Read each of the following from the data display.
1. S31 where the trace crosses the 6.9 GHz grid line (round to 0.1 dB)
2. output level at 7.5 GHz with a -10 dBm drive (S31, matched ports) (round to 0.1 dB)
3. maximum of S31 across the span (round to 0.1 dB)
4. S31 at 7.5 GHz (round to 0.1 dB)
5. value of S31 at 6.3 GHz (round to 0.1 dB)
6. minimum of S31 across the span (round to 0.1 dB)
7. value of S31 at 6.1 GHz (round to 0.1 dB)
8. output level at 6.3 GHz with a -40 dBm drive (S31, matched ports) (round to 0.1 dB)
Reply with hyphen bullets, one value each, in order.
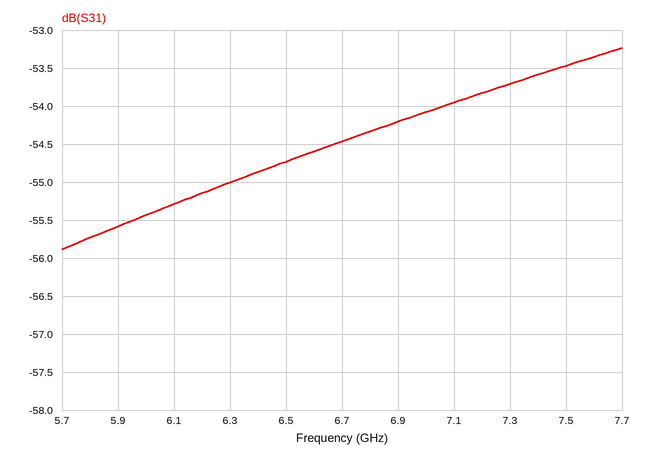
- -54.2 dB
- -63.5 dBm
- -53.2 dB
- -53.5 dB
- -55.0 dB
- -55.9 dB
- -55.3 dB
- -95.0 dBm
